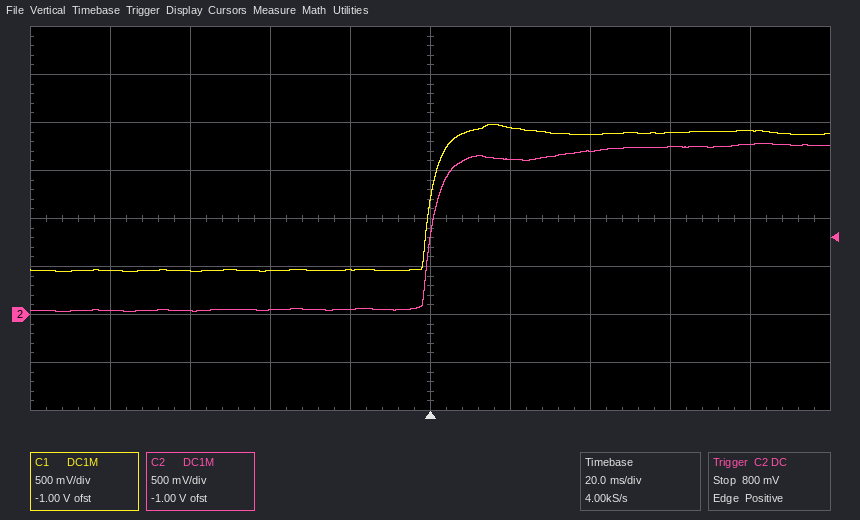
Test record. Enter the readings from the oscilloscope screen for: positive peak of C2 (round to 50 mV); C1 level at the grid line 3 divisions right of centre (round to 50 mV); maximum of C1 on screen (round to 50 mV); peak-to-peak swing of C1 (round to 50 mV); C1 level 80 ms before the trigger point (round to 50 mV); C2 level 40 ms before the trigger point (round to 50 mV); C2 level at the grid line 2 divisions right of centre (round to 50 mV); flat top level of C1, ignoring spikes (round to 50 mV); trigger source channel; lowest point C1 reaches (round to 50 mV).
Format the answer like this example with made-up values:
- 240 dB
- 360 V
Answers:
- 1.80 V
- 1.90 V
- 2.00 V
- 1.55 V
- 450 mV
- 50 mV
- 1.70 V
- 1.90 V
- C2
- 450 mV
